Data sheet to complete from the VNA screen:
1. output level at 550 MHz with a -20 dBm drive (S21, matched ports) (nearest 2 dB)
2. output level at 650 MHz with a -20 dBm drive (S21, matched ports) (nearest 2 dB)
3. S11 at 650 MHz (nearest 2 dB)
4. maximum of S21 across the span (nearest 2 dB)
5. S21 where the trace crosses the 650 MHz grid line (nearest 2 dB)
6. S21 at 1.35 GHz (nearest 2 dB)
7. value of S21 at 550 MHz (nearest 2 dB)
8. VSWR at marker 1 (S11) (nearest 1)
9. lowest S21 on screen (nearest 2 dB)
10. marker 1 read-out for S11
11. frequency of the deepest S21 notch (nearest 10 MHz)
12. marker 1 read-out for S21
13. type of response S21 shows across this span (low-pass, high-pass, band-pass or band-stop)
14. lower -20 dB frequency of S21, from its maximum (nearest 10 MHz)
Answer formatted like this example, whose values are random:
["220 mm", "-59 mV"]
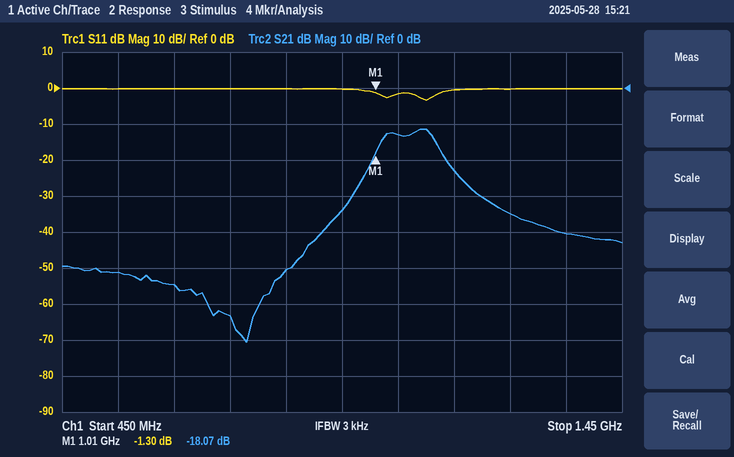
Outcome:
["-72 dBm", "-74 dBm", "0 dB", "-12 dB", "-54 dB", "-40 dB", "-52 dB", "13", "-70 dB", "-1.30 dB", "780 MHz", "-18.07 dB", "band-pass", "960 MHz"]
